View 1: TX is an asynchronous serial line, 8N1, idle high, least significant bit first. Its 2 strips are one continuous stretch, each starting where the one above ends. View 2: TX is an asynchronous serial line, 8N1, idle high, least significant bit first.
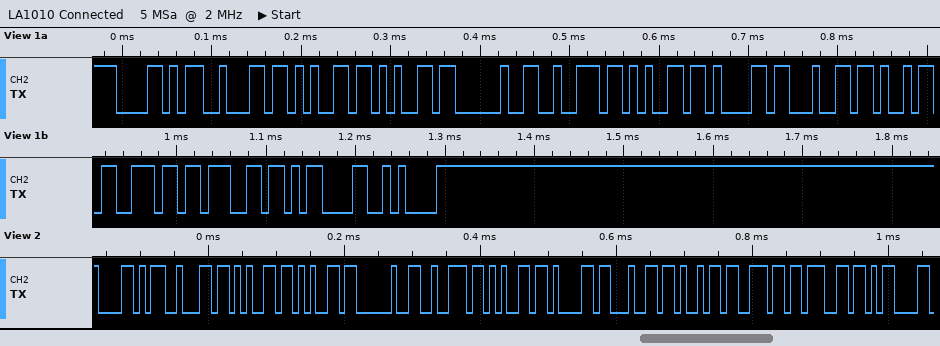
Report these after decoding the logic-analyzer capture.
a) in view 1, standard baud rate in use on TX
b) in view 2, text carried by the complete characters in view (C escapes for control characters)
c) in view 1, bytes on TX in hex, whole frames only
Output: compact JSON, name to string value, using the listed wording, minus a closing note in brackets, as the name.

{"in view 1, standard baud rate in use on TX": "115200 baud", "in view 2, text carried by the complete characters in view": "\"Xbee reading\\r\"", "in view 1, bytes on TX in hex, whole frames only": "58 62 65 65 20 72 65 61 64 69 6E 67 0D 0A"}
